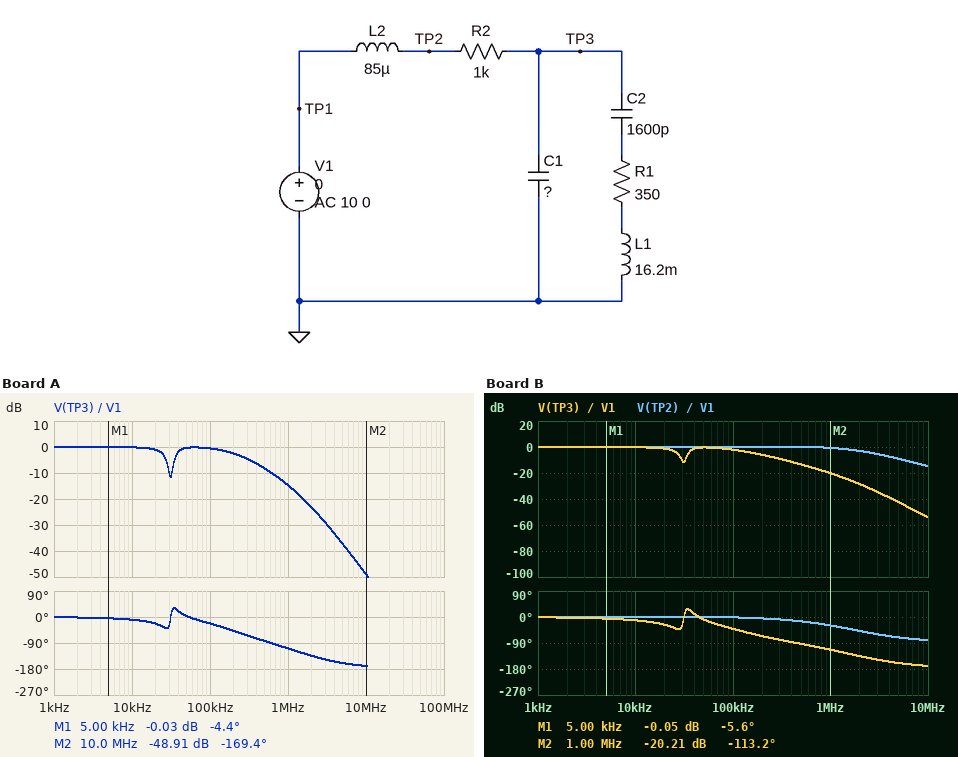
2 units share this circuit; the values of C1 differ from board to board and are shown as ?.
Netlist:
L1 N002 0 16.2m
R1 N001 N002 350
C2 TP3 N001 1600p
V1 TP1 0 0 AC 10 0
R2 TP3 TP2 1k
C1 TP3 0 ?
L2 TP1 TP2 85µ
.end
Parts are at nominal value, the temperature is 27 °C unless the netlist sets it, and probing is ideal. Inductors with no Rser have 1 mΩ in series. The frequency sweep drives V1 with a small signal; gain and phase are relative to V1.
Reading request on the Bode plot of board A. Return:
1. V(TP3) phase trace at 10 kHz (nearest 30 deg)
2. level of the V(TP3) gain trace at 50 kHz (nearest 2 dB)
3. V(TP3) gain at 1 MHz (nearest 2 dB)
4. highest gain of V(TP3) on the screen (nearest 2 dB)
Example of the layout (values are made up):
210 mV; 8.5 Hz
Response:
0 deg; 0 dB; -14 dB; 0 dB
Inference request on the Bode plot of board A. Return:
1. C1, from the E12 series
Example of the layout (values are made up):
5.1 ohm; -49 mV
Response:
820 pF
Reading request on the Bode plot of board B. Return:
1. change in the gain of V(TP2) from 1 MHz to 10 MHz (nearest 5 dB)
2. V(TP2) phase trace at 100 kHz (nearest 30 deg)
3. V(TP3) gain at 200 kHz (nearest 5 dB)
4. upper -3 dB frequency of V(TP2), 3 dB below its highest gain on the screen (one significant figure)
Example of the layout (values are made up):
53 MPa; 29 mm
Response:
-15 dB; 0 deg; -5 dB; 2 MHz
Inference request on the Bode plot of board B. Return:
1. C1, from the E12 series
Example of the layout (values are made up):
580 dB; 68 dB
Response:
1.5 nF
